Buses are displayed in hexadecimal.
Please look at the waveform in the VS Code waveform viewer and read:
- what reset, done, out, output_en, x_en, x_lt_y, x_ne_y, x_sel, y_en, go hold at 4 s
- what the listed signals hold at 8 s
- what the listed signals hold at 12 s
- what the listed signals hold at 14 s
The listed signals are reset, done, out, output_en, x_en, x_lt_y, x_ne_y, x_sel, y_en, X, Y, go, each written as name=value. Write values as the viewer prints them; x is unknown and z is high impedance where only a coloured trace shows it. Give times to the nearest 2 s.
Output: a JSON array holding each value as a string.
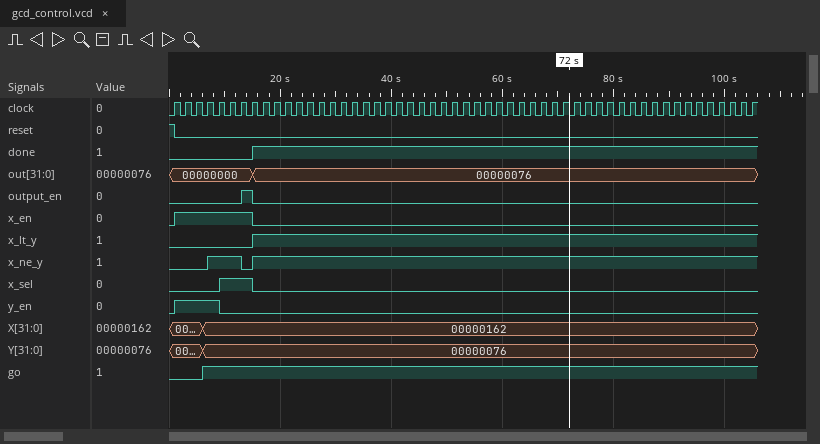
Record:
["reset=0, done=0, out=00000000, output_en=0, x_en=1, x_lt_y=0, x_ne_y=0, x_sel=0, y_en=1, go=0", "reset=0, done=0, out=00000000, output_en=0, x_en=1, x_lt_y=0, x_ne_y=1, x_sel=0, y_en=1, X=00000162, Y=00000076, go=1", "reset=0, done=0, out=00000000, output_en=0, x_en=1, x_lt_y=0, x_ne_y=1, x_sel=1, y_en=0, X=00000162, Y=00000076, go=1", "reset=0, done=0, out=00000000, output_en=1, x_en=1, x_lt_y=0, x_ne_y=0, x_sel=1, y_en=0, X=00000162, Y=00000076, go=1"]
